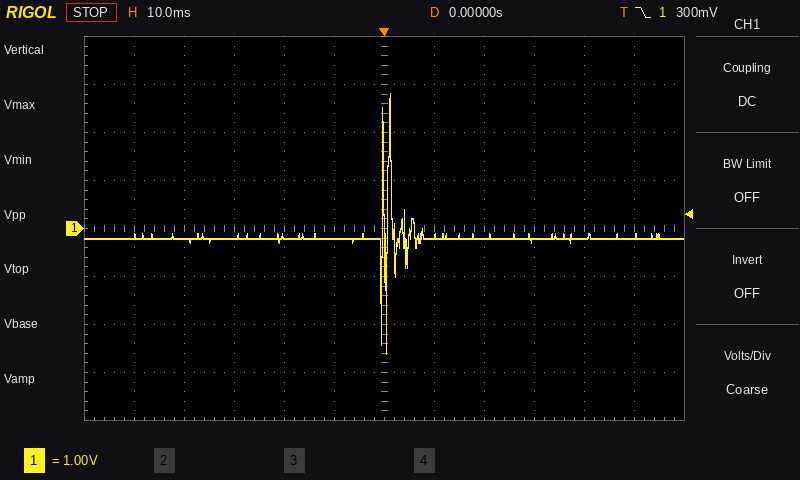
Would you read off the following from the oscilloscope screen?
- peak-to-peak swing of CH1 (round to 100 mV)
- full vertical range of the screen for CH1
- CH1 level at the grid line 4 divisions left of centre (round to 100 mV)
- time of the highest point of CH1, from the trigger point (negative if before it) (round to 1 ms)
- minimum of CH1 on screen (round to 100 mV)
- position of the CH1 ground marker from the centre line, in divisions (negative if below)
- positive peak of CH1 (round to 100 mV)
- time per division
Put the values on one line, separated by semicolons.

5.4 V; 8 V; -200 mV; +1 ms; -2.6 V; 0.0 div; 2.8 V; 10 ms
